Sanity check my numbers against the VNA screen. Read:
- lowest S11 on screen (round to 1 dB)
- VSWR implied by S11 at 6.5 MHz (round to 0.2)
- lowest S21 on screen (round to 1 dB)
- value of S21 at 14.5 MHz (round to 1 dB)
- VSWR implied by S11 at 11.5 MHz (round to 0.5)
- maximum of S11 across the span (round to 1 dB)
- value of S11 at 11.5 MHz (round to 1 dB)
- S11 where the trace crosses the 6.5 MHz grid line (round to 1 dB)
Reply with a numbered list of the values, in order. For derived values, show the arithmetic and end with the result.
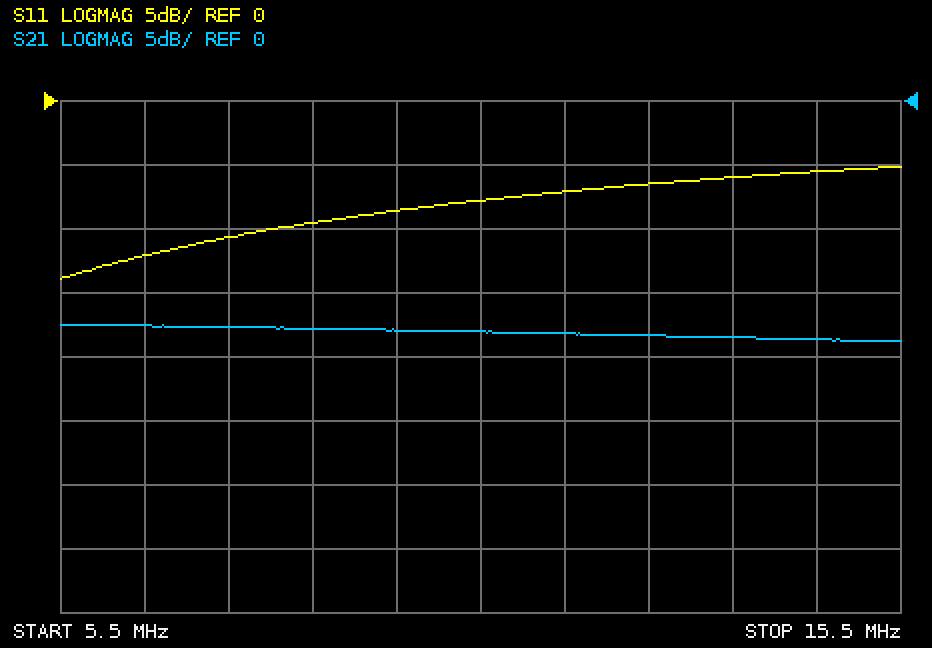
1. -14 dB
2. |Γ| = 10^(-12/20) = 0.2512; VSWR = (1 + 0.2512)/(1 − 0.2512) ≈ 1.67, so 1.6 to the nearest 0.2
3. -19 dB
4. -19 dB
5. |Γ| = 10^(-7/20) = 0.4467; VSWR = (1 + 0.4467)/(1 − 0.4467) ≈ 2.61, so 2.5 to the nearest 0.5
6. -5 dB
7. -7 dB
8. -12 dB
